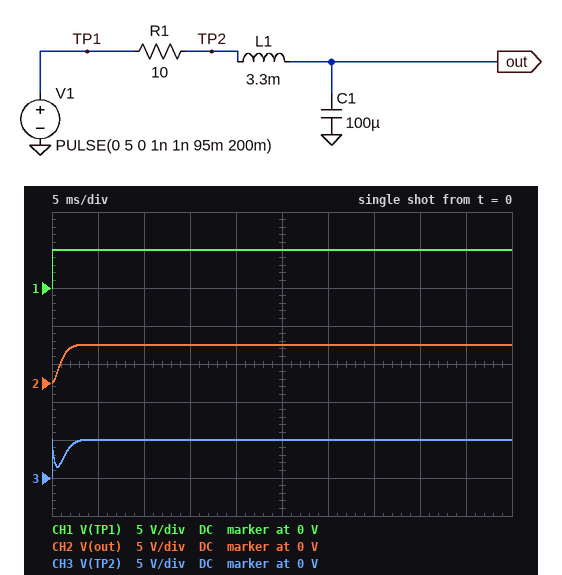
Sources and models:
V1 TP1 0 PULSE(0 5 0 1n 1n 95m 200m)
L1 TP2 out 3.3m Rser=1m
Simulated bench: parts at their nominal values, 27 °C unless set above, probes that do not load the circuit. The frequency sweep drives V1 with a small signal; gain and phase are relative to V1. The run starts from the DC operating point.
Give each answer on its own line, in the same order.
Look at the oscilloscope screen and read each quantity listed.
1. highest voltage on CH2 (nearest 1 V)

5 V
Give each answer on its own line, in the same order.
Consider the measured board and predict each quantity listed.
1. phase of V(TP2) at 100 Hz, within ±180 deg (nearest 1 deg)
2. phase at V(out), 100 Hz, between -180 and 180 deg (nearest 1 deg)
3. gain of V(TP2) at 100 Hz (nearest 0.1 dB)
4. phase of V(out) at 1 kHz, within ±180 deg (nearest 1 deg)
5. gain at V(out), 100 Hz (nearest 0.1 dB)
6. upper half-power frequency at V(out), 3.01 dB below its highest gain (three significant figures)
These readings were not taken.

-36 deg
-36 deg
-1.8 dB
-152 deg
-0.6 dB
216 Hz
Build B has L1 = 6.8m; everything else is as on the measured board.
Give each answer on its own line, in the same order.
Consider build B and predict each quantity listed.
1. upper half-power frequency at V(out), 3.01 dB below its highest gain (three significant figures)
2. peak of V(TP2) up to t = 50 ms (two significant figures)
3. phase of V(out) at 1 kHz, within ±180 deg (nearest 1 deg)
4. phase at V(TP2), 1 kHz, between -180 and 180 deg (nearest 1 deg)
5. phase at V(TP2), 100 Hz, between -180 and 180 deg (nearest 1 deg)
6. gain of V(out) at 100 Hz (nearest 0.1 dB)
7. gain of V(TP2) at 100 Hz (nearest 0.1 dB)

214 Hz
5.3 V
-166 deg
14 deg
-41 deg
0.3 dB
-2.4 dB
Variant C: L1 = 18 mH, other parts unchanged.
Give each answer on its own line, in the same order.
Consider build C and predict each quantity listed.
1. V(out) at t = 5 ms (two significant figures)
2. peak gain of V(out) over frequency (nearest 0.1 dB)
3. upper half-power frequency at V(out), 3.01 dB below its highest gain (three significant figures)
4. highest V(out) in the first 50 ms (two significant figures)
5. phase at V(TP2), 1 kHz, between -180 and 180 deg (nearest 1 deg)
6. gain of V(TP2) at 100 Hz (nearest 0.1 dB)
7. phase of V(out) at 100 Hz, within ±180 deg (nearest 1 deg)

6.3 V
3.2 dB
141 Hz
6.4 V
5 deg
-7.6 dB
-65 deg
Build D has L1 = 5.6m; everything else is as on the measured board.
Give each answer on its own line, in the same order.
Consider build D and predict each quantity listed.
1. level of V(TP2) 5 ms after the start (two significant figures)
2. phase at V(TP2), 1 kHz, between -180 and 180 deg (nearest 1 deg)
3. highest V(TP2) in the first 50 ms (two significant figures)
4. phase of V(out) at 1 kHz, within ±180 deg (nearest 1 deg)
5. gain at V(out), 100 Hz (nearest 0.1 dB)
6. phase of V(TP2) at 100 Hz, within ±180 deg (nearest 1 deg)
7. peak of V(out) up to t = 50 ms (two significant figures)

5.1 V
17 deg
5.2 V
-163 deg
0 dB
-39 deg
5.3 V
